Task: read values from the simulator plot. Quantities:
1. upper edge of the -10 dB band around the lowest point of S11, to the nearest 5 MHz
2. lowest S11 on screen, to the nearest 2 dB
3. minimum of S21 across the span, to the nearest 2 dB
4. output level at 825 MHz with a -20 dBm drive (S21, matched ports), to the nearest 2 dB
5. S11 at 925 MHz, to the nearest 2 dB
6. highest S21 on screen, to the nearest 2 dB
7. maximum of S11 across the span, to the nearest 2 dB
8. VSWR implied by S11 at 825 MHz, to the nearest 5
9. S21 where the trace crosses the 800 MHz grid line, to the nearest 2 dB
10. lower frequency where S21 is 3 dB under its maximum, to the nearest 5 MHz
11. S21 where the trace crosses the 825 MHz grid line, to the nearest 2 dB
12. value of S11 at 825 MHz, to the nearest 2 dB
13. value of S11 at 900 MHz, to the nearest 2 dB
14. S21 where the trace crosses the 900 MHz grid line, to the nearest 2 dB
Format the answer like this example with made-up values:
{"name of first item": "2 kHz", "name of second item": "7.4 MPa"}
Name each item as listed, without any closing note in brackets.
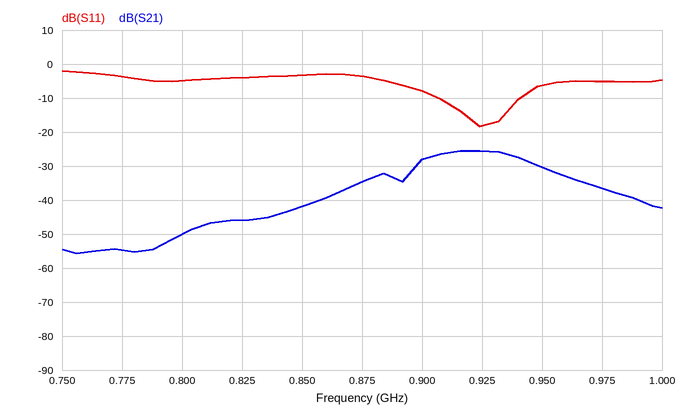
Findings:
{"upper edge of the -10 dB band around the lowest point of S11, to the nearest 5 MHz": "940 MHz", "lowest S11 on screen, to the nearest 2 dB": "-18 dB", "minimum of S21 across the span, to the nearest 2 dB": "-56 dB", "output level at 825 MHz with a -20 dBm drive (S21, matched ports), to the nearest 2 dB": "-66 dBm", "S11 at 925 MHz, to the nearest 2 dB": "-18 dB", "highest S21 on screen, to the nearest 2 dB": "-26 dB", "maximum of S11 across the span, to the nearest 2 dB": "-2 dB", "VSWR implied by S11 at 825 MHz, to the nearest 5": "5", "S21 where the trace crosses the 800 MHz grid line, to the nearest 2 dB": "-50 dB", "lower frequency where S21 is 3 dB under its maximum, to the nearest 5 MHz": "900 MHz", "S21 where the trace crosses the 825 MHz grid line, to the nearest 2 dB": "-46 dB", "value of S11 at 825 MHz, to the nearest 2 dB": "-4 dB", "value of S11 at 900 MHz, to the nearest 2 dB": "-8 dB", "S21 where the trace crosses the 900 MHz grid line, to the nearest 2 dB": "-28 dB"}
